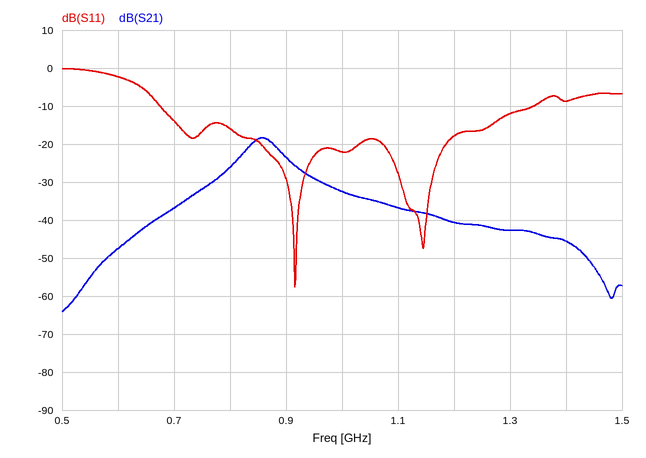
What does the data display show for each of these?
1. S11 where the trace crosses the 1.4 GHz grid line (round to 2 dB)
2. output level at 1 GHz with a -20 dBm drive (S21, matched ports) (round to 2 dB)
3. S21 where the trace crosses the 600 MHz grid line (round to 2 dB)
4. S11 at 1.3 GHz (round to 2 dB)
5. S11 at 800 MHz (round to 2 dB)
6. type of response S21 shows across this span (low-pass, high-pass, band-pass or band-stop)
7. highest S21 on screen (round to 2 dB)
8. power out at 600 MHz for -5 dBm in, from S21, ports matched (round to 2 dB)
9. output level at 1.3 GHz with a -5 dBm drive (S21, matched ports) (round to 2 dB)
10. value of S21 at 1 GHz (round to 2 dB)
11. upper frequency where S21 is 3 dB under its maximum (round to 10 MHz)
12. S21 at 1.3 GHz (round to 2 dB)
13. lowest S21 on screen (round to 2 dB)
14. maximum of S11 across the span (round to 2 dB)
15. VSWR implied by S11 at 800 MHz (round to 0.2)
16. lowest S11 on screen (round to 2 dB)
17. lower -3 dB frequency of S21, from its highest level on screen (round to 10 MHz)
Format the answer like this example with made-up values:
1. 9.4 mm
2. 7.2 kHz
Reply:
1. -8 dB
2. -52 dBm
3. -48 dB
4. -12 dB
5. -16 dB
6. band-pass
7. -18 dB
8. -52 dBm
9. -48 dBm
10. -32 dB
11. 890 MHz
12. -42 dB
13. -64 dB
14. 0 dB
15. 1.4
16. -58 dB
17. 830 MHz
